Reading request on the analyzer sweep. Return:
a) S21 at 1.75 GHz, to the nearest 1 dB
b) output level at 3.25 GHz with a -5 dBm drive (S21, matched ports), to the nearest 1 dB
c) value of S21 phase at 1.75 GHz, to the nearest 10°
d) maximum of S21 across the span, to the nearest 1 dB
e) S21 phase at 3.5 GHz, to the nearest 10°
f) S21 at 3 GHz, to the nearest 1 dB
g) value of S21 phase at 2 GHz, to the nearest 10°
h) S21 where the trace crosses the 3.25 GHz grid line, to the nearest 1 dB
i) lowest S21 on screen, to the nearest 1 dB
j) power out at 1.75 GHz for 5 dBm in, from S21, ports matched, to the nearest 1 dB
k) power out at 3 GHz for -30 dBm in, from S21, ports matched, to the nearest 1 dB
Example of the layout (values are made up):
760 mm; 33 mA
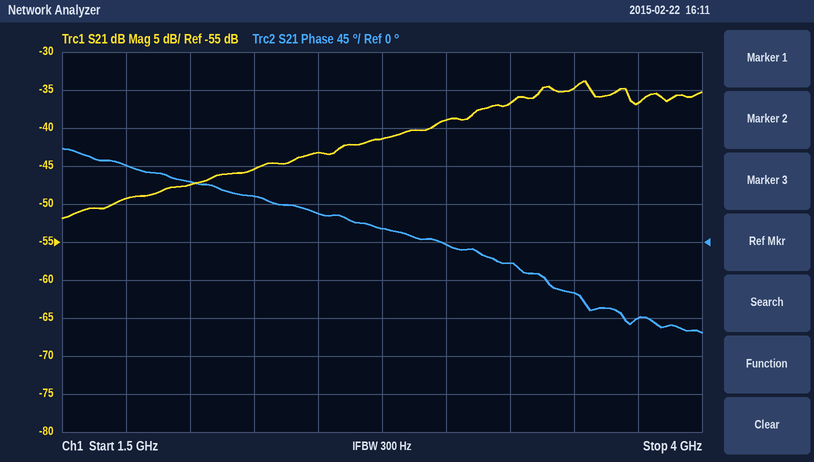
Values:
-49 dB; -42 dBm; 90°; -34 dB; -60°; -39 dB; 70°; -37 dB; -52 dB; -44 dBm; -69 dBm
